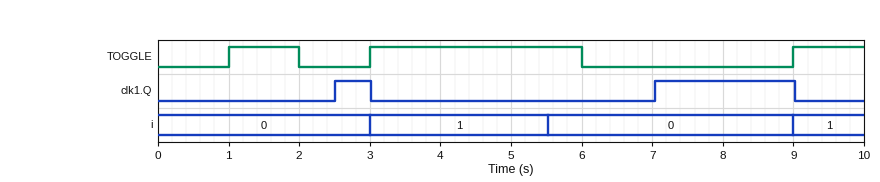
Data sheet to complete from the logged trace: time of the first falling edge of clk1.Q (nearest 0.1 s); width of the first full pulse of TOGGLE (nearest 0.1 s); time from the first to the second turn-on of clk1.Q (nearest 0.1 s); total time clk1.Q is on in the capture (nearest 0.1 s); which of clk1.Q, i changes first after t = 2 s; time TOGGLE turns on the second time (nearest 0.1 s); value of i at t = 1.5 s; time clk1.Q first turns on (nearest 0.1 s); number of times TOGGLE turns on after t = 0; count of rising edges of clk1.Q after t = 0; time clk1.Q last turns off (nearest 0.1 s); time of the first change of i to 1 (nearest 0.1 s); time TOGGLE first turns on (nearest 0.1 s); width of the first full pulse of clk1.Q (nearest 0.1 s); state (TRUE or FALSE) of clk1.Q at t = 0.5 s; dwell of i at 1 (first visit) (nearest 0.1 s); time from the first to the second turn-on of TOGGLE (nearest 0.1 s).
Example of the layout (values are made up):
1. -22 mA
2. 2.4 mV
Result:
1. 3.0 s
2. 1.0 s
3. 4.5 s
4. 2.5 s
5. clk1.Q
6. 3.0 s
7. 0
8. 2.5 s
9. 3
10. 2
11. 9.0 s
12. 3.0 s
13. 1.0 s
14. 0.5 s
15. FALSE
16. 2.5 s
17. 2.0 s
